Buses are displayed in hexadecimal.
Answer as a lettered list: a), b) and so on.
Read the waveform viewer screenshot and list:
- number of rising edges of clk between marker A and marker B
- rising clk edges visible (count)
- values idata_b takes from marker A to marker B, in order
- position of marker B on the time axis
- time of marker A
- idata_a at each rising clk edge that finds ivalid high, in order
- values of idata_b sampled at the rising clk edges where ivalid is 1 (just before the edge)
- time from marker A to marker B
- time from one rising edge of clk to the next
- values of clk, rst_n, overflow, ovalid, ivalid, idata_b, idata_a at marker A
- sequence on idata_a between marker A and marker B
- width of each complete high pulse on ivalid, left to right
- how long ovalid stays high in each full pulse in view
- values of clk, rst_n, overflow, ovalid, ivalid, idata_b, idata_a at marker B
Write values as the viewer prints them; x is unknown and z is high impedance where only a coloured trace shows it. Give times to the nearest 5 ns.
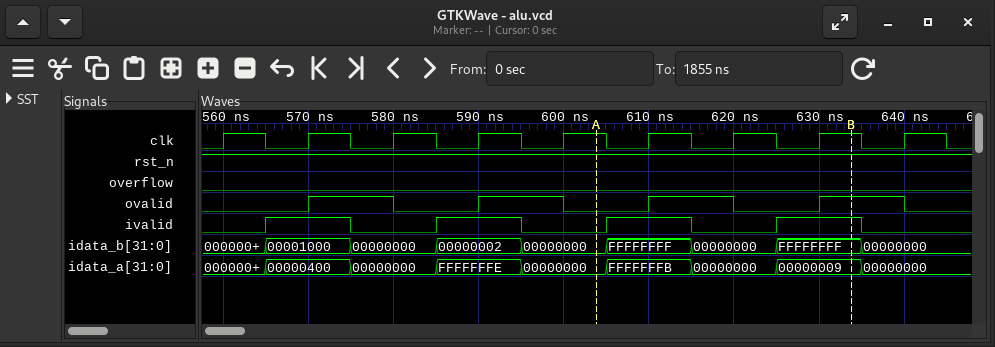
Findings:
a) 3
b) 9
c) 00000000, FFFFFFFF, 00000000, FFFFFFFF
d) 635 ns
e) 605 ns
f) 00000400, FFFFFFFE, FFFFFFFB, 00000009
g) 00001000, 00000002, FFFFFFFF, FFFFFFFF
h) 30 ns
i) 10 ns
j) clk=1, rst_n=1, overflow=0, ovalid=0, ivalid=0, idata_b=00000000, idata_a=00000000
k) 00000000, FFFFFFFB, 00000000, 00000009
l) 10 ns, 10 ns, 10 ns, 10 ns
m) 10 ns, 10 ns, 10 ns, 10 ns
n) clk=1, rst_n=1, overflow=0, ovalid=1, ivalid=1, idata_b=FFFFFFFF, idata_a=00000009
